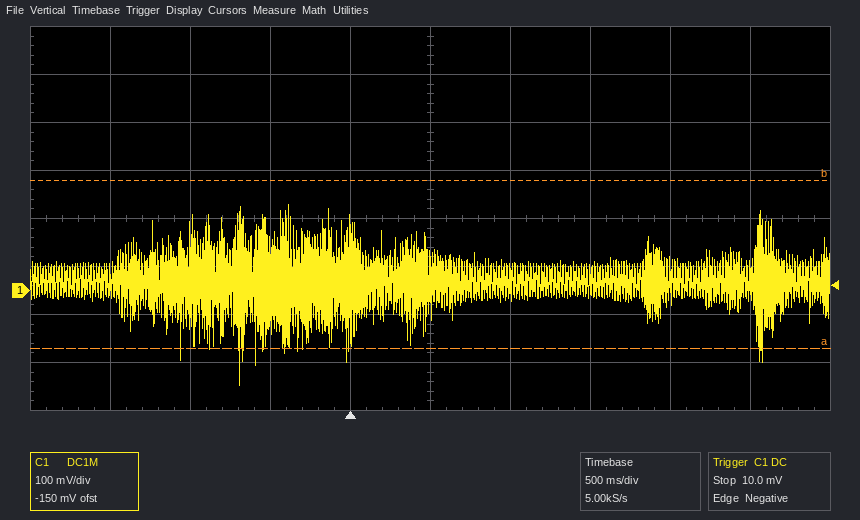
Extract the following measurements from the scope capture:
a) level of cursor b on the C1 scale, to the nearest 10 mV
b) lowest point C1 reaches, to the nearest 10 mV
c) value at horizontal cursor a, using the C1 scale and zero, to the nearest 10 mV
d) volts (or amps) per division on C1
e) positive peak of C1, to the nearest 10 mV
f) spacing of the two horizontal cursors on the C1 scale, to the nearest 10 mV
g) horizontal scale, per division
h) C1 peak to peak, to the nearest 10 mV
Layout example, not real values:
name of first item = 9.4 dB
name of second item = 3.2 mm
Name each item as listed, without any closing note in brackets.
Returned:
level of cursor b on the C1 scale, to the nearest 10 mV = 230 mV
lowest point C1 reaches, to the nearest 10 mV = -200 mV
value at horizontal cursor a, using the C1 scale and zero, to the nearest 10 mV = -120 mV
volts (or amps) per division on C1 = 100 mV
positive peak of C1, to the nearest 10 mV = 180 mV
spacing of the two horizontal cursors on the C1 scale, to the nearest 10 mV = 350 mV
horizontal scale, per division = 500 ms
C1 peak to peak, to the nearest 10 mV = 380 mV
